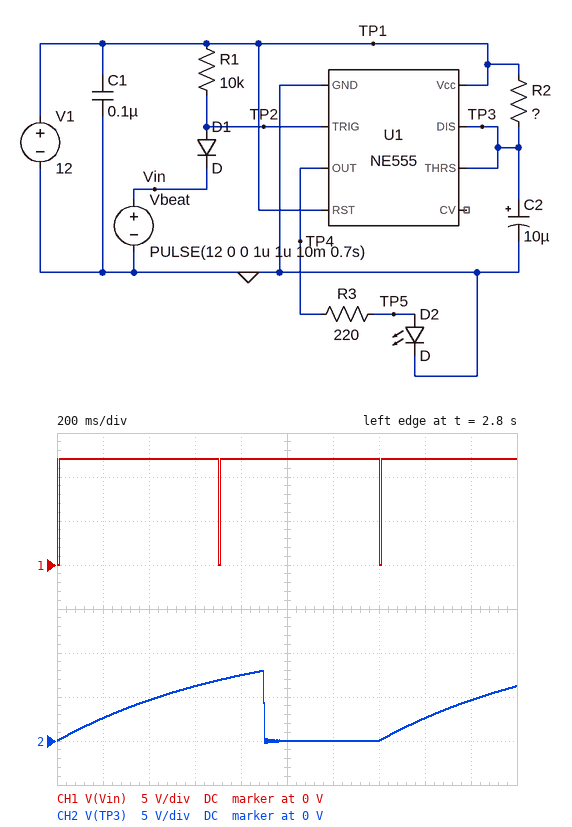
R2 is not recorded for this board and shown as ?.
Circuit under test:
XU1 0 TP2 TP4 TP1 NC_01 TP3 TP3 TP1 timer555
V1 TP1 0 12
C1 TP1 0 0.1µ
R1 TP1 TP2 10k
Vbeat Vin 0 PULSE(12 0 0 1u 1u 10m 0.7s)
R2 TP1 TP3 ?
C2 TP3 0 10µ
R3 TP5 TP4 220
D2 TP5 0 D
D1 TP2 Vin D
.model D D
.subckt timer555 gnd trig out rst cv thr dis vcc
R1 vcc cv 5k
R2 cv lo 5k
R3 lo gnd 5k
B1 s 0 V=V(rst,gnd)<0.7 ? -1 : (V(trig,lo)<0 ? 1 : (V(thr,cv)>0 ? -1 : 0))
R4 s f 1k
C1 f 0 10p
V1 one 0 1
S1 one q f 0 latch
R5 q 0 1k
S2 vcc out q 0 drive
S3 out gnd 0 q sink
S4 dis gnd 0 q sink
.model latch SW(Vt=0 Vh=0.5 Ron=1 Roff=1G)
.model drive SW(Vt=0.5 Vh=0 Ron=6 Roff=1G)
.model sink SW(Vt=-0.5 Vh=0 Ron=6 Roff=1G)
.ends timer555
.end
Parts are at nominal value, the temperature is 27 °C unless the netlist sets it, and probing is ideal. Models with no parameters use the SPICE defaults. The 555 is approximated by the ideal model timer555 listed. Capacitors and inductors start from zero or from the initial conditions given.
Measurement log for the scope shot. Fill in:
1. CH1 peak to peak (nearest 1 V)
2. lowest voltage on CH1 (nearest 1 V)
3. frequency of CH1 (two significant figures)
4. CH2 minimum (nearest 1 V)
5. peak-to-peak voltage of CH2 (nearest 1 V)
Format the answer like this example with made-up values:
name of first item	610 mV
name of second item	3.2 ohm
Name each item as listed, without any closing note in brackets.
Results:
CH1 peak to peak	12 V
lowest voltage on CH1	0 V
frequency of CH1	1.4 Hz
CH2 minimum	0 V
peak-to-peak voltage of CH2	8 V
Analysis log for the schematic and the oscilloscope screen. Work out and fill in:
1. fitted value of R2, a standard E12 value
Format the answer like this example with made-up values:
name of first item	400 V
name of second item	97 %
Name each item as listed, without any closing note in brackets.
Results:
fitted value of R2, a standard E12 value	82 kΩ
